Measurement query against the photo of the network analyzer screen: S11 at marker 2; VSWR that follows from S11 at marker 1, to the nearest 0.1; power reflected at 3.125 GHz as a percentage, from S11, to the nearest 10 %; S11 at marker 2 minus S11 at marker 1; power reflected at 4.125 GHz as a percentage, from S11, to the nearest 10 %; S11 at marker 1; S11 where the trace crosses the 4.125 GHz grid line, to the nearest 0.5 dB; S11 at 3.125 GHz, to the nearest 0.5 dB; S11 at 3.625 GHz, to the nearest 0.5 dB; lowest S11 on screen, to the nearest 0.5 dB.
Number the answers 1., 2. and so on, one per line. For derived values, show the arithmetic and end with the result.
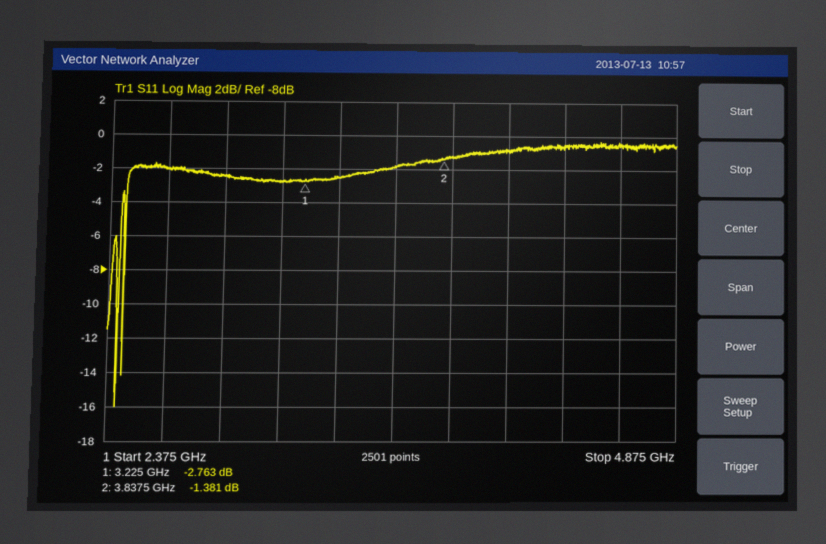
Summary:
1. -1.381 dB
2. (1 + 0.7275)/(1 − 0.7275) ≈ 6.3
3. 10^(-3/10) ≈ 50 %
4. -1.381 − (-2.763) = 1.382 dB
5. 10^(-1/10) ≈ 79.4 %, so 80 % to the nearest 10 %
6. -2.763 dB
7. -1.0 dB
8. -3.0 dB
9. -2.0 dB
10. -16.0 dB
